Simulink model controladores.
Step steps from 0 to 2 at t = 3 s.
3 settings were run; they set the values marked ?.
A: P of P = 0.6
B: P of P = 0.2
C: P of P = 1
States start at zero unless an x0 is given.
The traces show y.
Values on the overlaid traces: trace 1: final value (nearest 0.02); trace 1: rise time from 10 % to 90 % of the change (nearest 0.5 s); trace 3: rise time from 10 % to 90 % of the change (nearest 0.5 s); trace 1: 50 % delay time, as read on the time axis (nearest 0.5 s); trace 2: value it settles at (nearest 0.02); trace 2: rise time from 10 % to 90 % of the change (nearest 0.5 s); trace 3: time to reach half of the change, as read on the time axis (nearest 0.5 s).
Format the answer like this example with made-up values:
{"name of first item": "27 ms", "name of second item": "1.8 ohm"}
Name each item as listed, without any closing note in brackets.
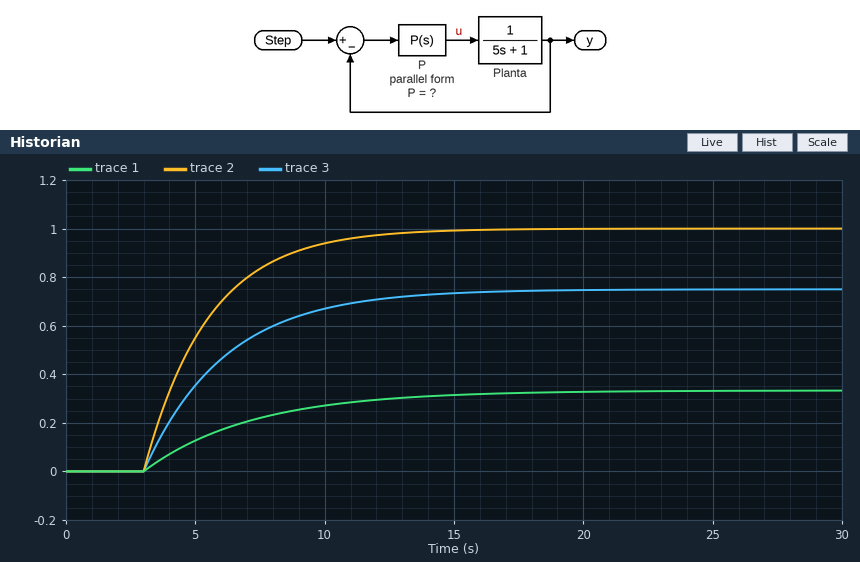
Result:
{"trace 1: final value": "0.34", "trace 1: rise time from 10 % to 90 % of the change": "9.0 s", "trace 3: rise time from 10 % to 90 % of the change": "7.0 s", "trace 1: 50 % delay time, as read on the time axis": "6.0 s", "trace 2: value it settles at": "1.00", "trace 2: rise time from 10 % to 90 % of the change": "5.5 s", "trace 3: time to reach half of the change, as read on the time axis": "5.0 s"}
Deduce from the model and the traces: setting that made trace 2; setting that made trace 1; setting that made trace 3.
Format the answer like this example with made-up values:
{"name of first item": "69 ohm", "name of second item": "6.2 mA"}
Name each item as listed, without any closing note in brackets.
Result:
{"setting that made trace 2": "C", "setting that made trace 1": "B", "setting that made trace 3": "A"}
